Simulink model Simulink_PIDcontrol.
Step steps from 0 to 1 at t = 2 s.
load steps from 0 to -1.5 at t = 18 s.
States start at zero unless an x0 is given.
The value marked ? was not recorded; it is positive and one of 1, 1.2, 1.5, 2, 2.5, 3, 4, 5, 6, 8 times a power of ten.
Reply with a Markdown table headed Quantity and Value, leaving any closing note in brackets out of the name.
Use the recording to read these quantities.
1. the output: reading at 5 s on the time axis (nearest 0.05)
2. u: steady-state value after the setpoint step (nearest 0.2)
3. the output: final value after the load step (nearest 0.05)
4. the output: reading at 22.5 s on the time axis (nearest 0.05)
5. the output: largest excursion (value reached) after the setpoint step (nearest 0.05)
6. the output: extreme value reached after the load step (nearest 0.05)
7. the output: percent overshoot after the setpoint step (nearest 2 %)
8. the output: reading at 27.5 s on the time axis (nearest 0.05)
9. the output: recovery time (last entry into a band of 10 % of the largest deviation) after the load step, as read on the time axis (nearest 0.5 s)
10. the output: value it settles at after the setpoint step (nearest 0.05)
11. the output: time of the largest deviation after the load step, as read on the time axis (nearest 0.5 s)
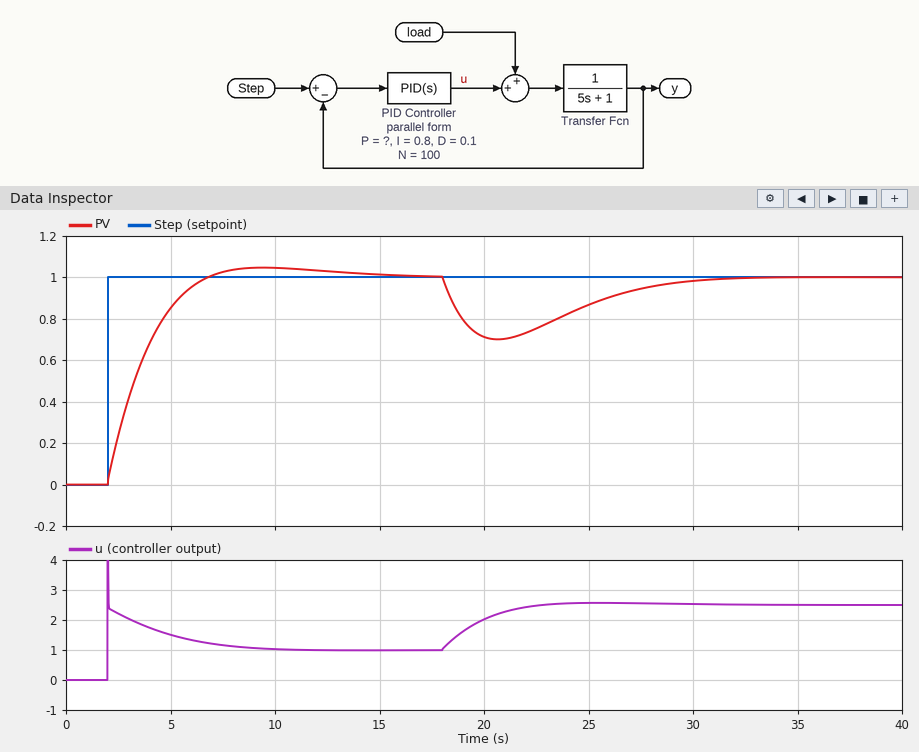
| Quantity | Value |
|---|---|
| the output: reading at 5 s on the time axis | 0.85 |
| u: steady-state value after the setpoint step | 1.0 |
| the output: final value after the load step | 1.00 |
| the output: reading at 22.5 s on the time axis | 0.75 |
| the output: largest excursion (value reached) after the setpoint step | 1.05 |
| the output: extreme value reached after the load step | 0.70 |
| the output: percent overshoot after the setpoint step | 4 % |
| the output: reading at 27.5 s on the time axis | 0.95 |
| the output: recovery time (last entry into a band of 10 % of the largest deviation) after the load step, as read on the time axis | 29.0 s |
| the output: value it settles at after the setpoint step | 1.00 |
| the output: time of the largest deviation after the load step, as read on the time axis | 20.5 s |
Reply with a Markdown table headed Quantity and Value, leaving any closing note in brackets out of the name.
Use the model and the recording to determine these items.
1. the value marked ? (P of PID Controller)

| Quantity | Value |
|---|---|
| the value marked ? | 2.5 |
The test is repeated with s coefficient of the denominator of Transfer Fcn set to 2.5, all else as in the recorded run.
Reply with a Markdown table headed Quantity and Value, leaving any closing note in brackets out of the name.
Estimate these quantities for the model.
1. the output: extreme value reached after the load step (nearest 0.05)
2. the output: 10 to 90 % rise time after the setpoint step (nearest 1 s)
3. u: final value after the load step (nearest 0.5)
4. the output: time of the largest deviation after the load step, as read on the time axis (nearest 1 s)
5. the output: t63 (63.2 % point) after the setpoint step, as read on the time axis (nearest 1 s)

| Quantity | Value |
|---|---|
| the output: extreme value reached after the load step | 0.65 |
| the output: 10 to 90 % rise time after the setpoint step | 3 s |
| u: final value after the load step | 2.5 |
| the output: time of the largest deviation after the load step, as read on the time axis | 20 s |
| the output: t63 (63.2 % point) after the setpoint step, as read on the time axis | 3 s |
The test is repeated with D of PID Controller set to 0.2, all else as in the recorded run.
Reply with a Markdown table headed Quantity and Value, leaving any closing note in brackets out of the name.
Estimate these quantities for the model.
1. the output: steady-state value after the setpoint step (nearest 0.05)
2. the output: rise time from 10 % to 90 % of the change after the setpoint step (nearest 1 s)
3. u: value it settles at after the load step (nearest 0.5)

| Quantity | Value |
|---|---|
| the output: steady-state value after the setpoint step | 1.00 |
| the output: rise time from 10 % to 90 % of the change after the setpoint step | 3 s |
| u: value it settles at after the load step | 2.5 |
